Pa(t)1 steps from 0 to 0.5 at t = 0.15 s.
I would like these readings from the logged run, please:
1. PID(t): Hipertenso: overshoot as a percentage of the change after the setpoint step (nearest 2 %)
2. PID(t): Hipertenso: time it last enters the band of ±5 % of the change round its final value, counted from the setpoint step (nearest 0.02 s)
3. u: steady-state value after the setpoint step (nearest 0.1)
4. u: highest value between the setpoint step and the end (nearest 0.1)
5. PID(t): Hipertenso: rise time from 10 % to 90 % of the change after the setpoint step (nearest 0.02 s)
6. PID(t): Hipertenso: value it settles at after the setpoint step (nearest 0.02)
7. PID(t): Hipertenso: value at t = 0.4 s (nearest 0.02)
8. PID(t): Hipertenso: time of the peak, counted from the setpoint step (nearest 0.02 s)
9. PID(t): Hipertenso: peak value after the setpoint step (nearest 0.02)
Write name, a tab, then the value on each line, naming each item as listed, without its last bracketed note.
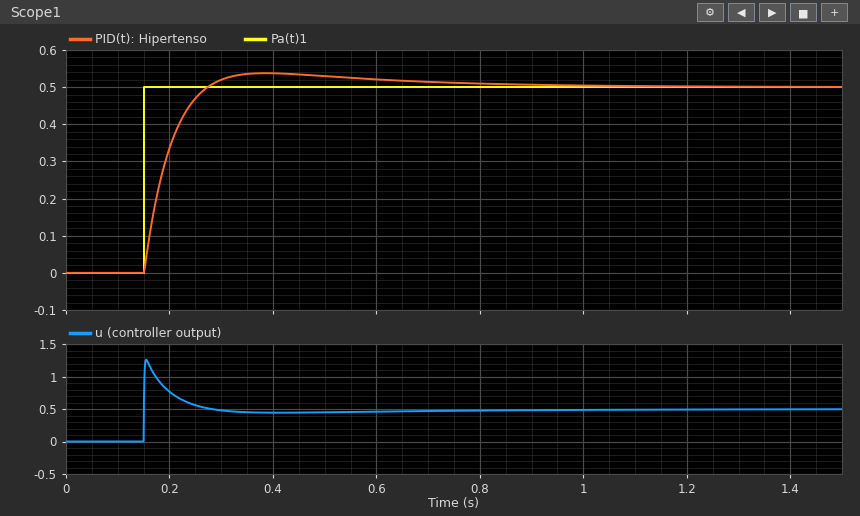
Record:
PID(t): Hipertenso: overshoot as a percentage of the change after the setpoint step	8 %
PID(t): Hipertenso: time it last enters the band of ±5 % of the change round its final value, counted from the setpoint step	0.40 s
u: steady-state value after the setpoint step	0.5
u: highest value between the setpoint step and the end	1.3
PID(t): Hipertenso: rise time from 10 % to 90 % of the change after the setpoint step	0.08 s
PID(t): Hipertenso: value it settles at after the setpoint step	0.50
PID(t): Hipertenso: value at t = 0.4 s	0.54
PID(t): Hipertenso: time of the peak, counted from the setpoint step	0.24 s
PID(t): Hipertenso: peak value after the setpoint step	0.54
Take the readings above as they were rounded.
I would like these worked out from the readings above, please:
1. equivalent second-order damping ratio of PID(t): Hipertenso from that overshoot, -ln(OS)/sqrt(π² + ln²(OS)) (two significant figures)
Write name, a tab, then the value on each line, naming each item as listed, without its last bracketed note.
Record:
equivalent second-order damping ratio of PID(t): Hipertenso from that overshoot, -ln(OS)/sqrt(π² + ln²(OS))	0.63
